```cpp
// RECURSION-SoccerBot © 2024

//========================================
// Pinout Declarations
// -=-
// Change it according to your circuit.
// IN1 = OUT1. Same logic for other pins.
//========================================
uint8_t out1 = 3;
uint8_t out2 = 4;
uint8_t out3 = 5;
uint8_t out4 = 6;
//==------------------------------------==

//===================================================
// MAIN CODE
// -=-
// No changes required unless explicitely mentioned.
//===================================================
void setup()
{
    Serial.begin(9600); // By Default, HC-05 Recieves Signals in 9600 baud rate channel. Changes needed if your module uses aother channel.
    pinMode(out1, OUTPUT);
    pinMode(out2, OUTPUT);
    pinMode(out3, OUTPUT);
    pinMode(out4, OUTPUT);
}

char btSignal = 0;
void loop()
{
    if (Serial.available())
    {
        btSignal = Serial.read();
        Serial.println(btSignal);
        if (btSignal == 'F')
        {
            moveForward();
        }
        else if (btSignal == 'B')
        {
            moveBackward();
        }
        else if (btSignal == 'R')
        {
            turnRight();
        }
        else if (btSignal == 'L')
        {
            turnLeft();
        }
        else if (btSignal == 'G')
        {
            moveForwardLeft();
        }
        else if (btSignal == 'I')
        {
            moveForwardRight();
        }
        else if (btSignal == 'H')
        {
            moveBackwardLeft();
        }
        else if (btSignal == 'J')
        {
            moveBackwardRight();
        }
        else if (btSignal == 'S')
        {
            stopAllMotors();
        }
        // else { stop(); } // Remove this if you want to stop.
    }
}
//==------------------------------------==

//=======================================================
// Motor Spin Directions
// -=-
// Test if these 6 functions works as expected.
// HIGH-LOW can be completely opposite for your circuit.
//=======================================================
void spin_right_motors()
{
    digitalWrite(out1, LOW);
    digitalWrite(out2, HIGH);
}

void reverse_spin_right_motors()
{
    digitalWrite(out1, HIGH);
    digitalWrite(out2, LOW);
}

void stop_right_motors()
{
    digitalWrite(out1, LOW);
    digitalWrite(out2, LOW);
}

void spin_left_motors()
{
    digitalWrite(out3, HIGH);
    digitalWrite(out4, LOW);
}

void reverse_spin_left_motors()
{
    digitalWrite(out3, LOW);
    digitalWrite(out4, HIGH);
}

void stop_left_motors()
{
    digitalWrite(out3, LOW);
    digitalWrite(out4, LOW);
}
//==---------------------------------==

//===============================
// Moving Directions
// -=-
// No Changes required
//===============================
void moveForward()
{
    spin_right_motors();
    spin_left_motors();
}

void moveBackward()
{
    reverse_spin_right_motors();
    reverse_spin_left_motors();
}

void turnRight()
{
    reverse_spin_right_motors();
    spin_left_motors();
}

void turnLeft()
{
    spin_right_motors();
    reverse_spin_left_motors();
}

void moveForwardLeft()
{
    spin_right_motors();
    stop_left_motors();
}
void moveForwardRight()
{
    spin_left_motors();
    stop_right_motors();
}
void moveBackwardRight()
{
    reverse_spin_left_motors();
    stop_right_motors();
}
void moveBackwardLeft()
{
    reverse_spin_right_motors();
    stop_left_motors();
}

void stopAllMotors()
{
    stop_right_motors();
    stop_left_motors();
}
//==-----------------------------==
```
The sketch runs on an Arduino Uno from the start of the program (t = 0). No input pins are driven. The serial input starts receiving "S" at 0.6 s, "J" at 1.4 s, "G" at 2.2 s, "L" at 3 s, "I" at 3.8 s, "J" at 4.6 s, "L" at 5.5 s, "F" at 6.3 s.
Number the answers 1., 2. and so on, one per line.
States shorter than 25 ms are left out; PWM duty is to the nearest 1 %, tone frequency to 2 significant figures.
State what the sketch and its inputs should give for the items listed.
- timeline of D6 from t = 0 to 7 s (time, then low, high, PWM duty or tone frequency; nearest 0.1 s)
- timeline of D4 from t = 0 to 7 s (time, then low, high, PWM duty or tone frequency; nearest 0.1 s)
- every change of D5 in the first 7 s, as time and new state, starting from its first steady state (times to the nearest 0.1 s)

1. 0 s low; 1.4 s high; 2.2 s low; 3 s high; 3.8 s low; 4.6 s high; 6.3 s low
2. 0 s low; 2.2 s high; 3.8 s low; 5.5 s high
3. 0 s low; 3.8 s high; 4.6 s low; 6.3 s high
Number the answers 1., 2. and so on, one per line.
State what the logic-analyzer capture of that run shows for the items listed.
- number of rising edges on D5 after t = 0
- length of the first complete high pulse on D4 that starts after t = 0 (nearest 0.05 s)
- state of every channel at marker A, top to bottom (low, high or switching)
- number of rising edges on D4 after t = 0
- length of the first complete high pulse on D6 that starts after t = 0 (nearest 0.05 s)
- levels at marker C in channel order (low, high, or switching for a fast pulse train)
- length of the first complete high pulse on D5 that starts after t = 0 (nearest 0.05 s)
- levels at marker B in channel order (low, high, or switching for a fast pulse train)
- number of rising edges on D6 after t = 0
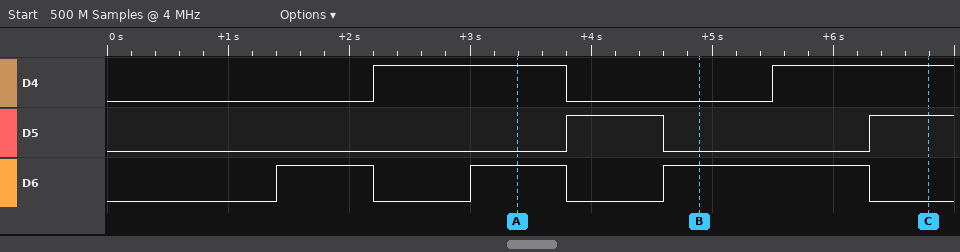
1. 2
2. 1.60 s
3. D4 high, D5 low, D6 high
4. 2
5. 0.80 s
6. D4 high, D5 high, D6 low
7. 0.80 s
8. D4 low, D5 low, D6 high
9. 3
